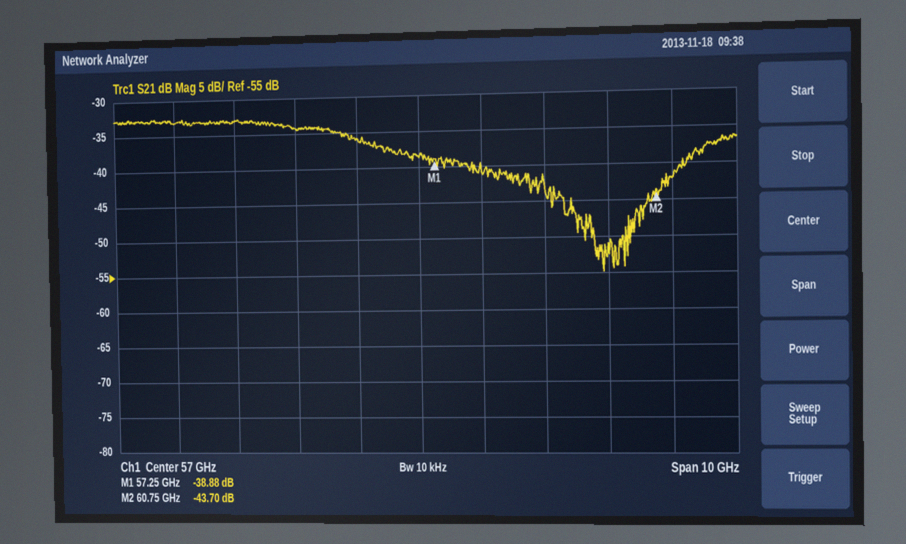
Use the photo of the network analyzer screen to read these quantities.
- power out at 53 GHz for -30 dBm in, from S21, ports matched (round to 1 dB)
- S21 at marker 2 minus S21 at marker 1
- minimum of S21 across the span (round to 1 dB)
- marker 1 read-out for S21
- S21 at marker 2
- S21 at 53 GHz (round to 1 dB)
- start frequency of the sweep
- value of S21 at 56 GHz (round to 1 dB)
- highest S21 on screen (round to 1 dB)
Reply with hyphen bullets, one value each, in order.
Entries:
- -63 dBm
- -4.82 dB
- -55 dB
- -38.88 dB
- -43.70 dB
- -33 dB
- 52 GHz
- -36 dB
- -33 dB
